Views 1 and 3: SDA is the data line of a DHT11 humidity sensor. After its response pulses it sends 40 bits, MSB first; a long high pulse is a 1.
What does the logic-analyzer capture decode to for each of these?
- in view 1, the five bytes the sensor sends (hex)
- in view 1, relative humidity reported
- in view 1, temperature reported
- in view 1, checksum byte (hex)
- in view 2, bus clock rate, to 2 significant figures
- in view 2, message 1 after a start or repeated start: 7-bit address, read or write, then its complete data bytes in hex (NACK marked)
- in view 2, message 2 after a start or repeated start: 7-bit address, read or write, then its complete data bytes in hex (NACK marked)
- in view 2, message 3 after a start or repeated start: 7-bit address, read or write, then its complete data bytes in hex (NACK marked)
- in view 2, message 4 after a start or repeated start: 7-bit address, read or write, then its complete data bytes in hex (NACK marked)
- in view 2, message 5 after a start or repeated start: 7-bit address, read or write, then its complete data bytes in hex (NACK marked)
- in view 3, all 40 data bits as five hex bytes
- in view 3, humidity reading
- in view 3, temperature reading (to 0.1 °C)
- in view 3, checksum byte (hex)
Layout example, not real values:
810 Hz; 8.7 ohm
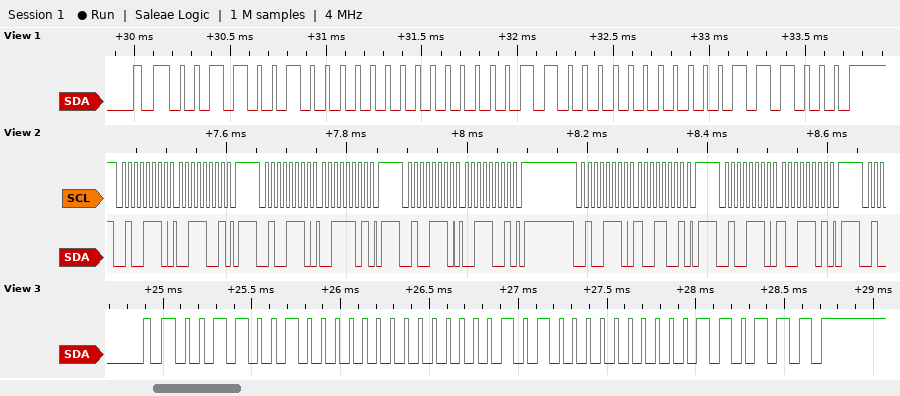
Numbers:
32 00 06 00 38; 50 %; 6.0 °C; 0x38; 100 kHz; 0x27 write: 39; 0x27 write: 3D; 0x27 write: 39; 0x27 write: 99; 0x27 write: 9D; 32 00 05 00 37; 50 %; 5.0 °C; 0x37
